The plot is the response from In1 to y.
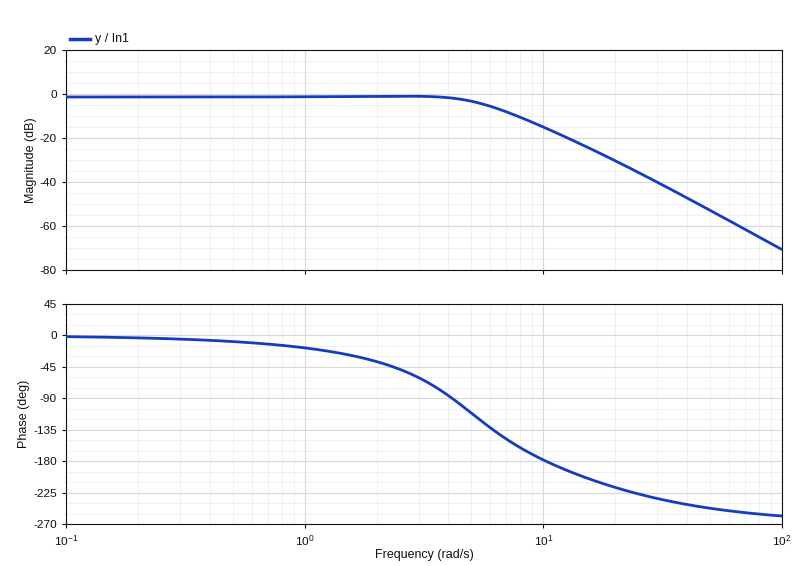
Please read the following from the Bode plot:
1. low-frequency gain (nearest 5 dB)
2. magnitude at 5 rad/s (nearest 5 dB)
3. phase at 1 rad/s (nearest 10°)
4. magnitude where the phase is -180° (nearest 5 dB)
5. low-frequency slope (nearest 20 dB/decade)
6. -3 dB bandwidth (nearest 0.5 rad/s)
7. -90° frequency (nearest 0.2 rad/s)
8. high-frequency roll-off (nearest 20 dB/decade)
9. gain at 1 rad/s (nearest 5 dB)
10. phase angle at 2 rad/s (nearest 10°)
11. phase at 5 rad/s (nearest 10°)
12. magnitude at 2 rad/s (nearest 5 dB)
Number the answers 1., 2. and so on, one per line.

1. 0 dB
2. -5 dB
3. -20°
4. -15 dB
5. 0 dB/decade
6. 5.5 rad/s
7. 4.2 rad/s
8. -60 dB/decade
9. 0 dB
10. -40°
11. -110°
12. 0 dB
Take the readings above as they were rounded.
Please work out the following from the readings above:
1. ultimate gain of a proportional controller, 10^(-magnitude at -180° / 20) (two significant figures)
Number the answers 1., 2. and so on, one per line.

1. 5.6
